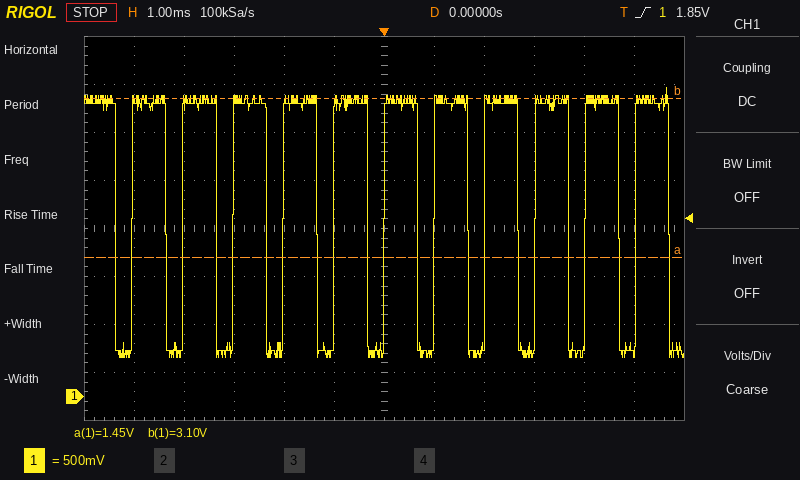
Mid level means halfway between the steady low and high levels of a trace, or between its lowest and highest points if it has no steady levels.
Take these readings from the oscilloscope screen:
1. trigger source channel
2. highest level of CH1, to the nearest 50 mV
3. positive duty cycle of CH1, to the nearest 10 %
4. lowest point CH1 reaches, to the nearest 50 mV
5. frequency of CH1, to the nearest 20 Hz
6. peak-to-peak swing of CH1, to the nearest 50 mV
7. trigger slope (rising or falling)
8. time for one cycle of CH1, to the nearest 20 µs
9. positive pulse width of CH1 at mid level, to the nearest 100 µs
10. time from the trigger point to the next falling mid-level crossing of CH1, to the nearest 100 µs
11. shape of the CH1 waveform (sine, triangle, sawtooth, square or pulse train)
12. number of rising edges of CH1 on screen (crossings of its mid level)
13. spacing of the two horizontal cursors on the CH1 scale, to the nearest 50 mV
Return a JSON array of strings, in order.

["CH1", "3.20 V", "70 %", "400 mV", "1.00 kHz", "2.80 V", "rising", "1.00 ms", "700 µs", "700 µs", "pulse train", "11", "1.65 V"]
